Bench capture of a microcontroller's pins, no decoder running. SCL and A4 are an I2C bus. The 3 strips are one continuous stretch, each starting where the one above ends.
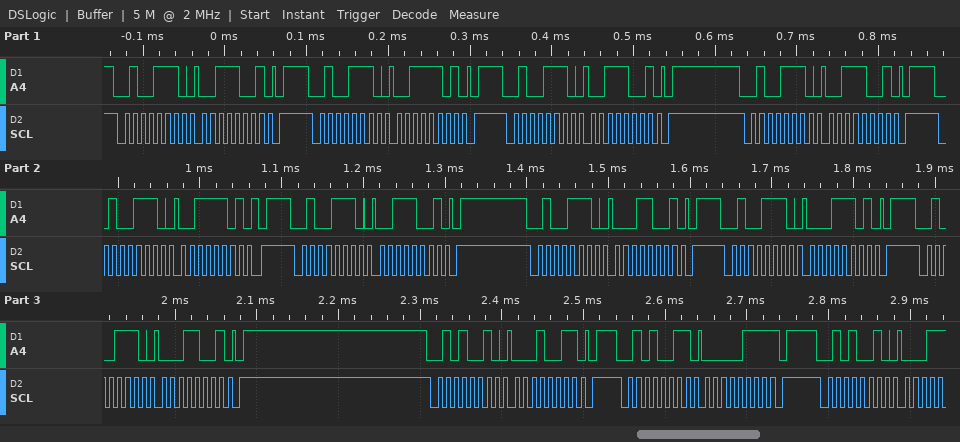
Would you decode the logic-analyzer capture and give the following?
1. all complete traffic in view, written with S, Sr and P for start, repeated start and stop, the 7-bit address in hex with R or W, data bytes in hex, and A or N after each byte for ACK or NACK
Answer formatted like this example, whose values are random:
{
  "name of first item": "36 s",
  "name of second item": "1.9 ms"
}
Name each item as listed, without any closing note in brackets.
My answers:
{
  "all complete traffic in view, written with S, Sr and P for start, repeated start and stop, the 7-bit address in hex with R or W, data bytes in hex, and A or N after each byte for ACK or NACK": "S 27W A 39 A P S 27W A 3D A P S 27W A 39 A P S 27W A 39 A P S 27W A 3D A P S 27W A 39 A P S 27W A 19 A P S 27W A 1D A P S 27W A 19 A P S 29W A 13 A P S 29R A 07 N P S 29W A"
}
